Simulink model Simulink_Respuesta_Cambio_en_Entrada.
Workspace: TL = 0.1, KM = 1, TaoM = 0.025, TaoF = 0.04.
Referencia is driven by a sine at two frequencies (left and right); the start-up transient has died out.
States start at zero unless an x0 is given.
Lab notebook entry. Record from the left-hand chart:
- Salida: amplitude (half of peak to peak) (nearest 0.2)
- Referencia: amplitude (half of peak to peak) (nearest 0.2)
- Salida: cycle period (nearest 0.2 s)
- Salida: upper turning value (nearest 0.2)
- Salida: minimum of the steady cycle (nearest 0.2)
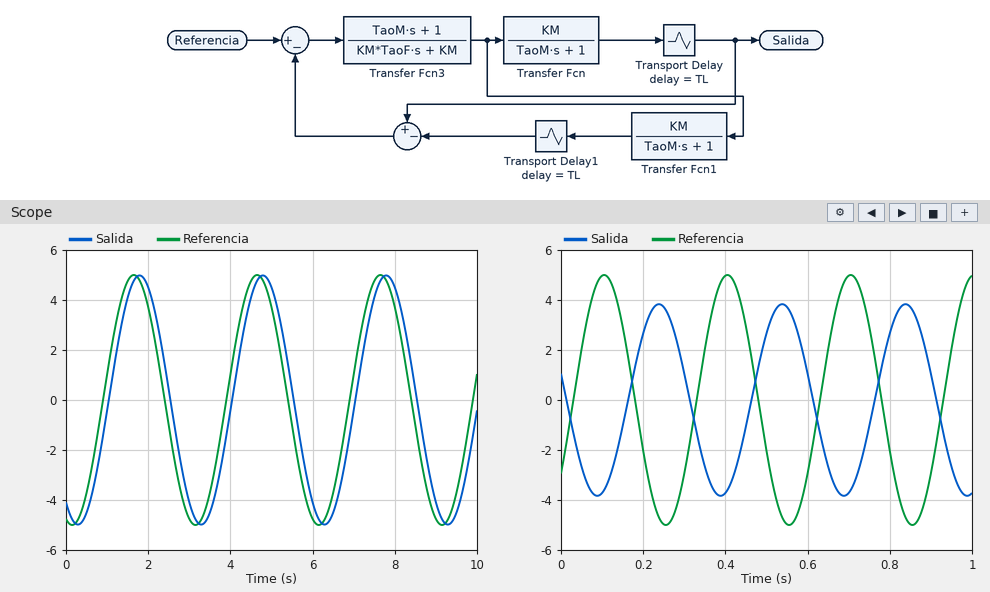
5.0
5.0
3.0 s
5.0
-5.0
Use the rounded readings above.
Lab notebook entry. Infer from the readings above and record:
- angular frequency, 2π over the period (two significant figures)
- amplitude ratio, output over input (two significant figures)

2.1 rad/s
1.0
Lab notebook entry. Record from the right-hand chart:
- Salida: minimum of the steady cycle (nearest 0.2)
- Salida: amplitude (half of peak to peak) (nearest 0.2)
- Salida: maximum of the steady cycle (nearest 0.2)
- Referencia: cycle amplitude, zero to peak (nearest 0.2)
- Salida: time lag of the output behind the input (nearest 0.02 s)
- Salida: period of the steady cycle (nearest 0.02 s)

-3.8
3.8
3.8
5.0
0.14 s
0.30 s
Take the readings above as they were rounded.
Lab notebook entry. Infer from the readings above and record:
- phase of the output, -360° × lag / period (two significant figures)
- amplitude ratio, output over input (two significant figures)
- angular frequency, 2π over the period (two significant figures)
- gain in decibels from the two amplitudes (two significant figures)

-170°
0.76
21 rad/s
-2.4 dB
